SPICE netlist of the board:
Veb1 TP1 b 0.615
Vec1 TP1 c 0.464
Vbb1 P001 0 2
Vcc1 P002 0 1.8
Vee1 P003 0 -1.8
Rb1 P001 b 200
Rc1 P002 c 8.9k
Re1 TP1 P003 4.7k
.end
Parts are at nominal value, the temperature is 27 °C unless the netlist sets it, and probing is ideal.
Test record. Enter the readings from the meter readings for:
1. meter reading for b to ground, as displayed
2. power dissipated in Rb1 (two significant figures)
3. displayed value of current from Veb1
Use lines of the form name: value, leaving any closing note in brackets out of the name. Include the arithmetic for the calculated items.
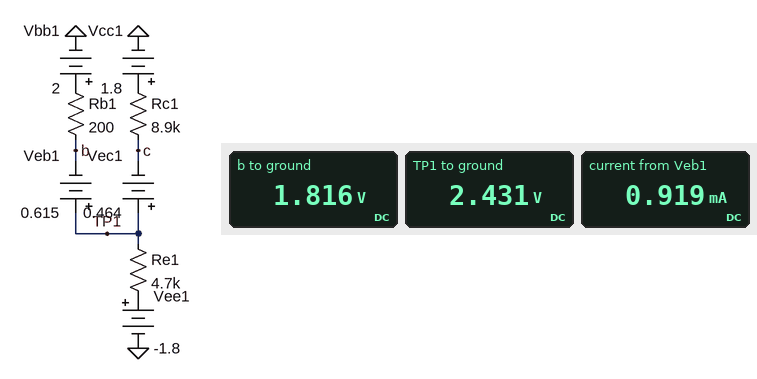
meter reading for b to ground, as displayed: 1.816 V
power dissipated in Rb1: (2 V - 1.816 V)^2 / 200 Ω = 170 µW
displayed value of current from Veb1: 0.919 mA
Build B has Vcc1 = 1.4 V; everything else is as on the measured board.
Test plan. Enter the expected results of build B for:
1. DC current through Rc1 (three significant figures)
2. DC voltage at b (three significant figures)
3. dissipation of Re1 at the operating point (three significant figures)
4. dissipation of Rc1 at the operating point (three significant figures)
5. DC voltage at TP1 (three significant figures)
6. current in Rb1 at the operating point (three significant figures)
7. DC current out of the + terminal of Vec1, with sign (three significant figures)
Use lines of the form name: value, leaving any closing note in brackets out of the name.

DC current through Rc1: 62.8 µA
DC voltage at b: 1.81 V
dissipation of Re1 at the operating point: 3.79 mW
dissipation of Rc1 at the operating point: 35.1 µW
DC voltage at TP1: 2.42 V
current in Rb1 at the operating point: 961 µA
DC current out of the + terminal of Vec1, with sign: -62.8 µA
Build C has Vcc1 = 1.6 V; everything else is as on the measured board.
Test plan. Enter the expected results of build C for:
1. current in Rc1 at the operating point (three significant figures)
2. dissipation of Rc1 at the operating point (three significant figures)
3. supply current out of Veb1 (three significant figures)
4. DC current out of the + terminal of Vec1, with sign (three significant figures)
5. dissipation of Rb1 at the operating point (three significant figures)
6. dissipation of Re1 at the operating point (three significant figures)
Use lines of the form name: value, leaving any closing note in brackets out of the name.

current in Rc1 at the operating point: 40.8 µA
dissipation of Rc1 at the operating point: 14.8 µW
supply current out of Veb1: 940 µA
DC current out of the + terminal of Vec1, with sign: -40.8 µA
dissipation of Rb1 at the operating point: 177 µW
dissipation of Re1 at the operating point: 3.80 mW
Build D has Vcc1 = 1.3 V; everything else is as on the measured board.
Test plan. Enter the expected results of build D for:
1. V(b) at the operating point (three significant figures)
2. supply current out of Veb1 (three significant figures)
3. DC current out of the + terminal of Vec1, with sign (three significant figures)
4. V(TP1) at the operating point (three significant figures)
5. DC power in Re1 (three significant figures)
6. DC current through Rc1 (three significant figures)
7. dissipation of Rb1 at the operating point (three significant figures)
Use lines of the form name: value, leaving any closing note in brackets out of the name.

V(b) at the operating point: 1.81 V
supply current out of Veb1: 972 µA
DC current out of the + terminal of Vec1, with sign: -73.8 µA
V(TP1) at the operating point: 2.42 V
DC power in Re1: 3.79 mW
DC current through Rc1: 73.8 µA
dissipation of Rb1 at the operating point: 189 µW
